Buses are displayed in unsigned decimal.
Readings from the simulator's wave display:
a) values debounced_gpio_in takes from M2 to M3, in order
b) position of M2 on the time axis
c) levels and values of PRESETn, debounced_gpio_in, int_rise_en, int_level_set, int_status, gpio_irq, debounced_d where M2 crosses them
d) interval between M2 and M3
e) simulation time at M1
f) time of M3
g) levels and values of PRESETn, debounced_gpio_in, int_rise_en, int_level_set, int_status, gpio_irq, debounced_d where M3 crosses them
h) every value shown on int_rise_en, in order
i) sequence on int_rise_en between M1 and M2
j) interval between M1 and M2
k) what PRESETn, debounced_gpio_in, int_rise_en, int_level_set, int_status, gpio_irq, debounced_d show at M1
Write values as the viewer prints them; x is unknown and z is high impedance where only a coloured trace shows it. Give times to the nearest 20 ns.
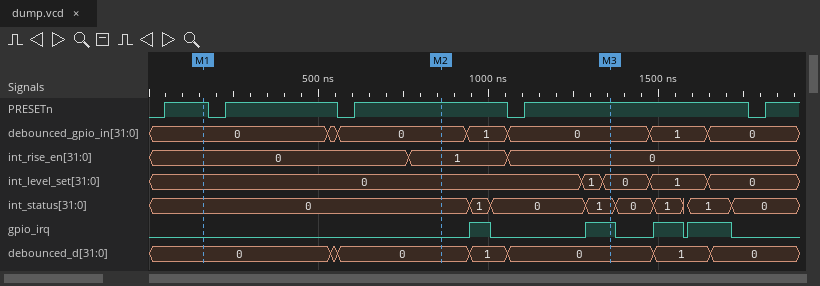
0, 1, 0
860 ns
PRESETn=1, debounced_gpio_in=0, int_rise_en=1, int_level_set=0, int_status=0, gpio_irq=0, debounced_d=0
500 ns
160 ns
1360 ns
PRESETn=1, debounced_gpio_in=0, int_rise_en=0, int_level_set=0, int_status=1, gpio_irq=1, debounced_d=0
0, 1, 0
0, 1
700 ns
PRESETn=1, debounced_gpio_in=0, int_rise_en=0, int_level_set=0, int_status=0, gpio_irq=0, debounced_d=0
